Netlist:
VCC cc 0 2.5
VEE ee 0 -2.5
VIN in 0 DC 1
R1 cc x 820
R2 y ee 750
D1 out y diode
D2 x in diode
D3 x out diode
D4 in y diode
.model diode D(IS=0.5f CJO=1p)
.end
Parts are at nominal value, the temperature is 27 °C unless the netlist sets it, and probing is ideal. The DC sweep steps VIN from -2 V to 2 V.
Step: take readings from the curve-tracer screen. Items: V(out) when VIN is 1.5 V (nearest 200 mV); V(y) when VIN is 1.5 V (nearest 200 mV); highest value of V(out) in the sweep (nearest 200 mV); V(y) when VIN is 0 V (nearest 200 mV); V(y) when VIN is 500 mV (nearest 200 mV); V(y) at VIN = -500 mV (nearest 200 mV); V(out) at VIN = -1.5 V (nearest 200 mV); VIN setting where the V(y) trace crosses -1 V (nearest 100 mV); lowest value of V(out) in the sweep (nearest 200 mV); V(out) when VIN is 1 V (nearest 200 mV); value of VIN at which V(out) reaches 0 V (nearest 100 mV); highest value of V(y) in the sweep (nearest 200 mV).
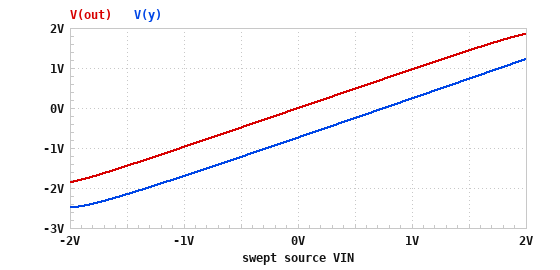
1.4 V
800 mV
1.8 V
-800 mV
-200 mV
-1.2 V
-1.4 V
-300 mV
-1.8 V
1.0 V
0 V
1.2 V
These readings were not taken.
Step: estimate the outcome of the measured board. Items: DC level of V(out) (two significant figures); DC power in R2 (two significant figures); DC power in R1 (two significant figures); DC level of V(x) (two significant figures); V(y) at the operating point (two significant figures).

970 mV
10 mW
800 µW
1.7 V
240 mV
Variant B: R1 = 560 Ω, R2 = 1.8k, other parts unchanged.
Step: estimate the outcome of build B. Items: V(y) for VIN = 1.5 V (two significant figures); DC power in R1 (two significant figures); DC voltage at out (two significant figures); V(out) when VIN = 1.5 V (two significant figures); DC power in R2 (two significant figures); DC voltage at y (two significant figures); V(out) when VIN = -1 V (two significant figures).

760 mV
1.1 mW
1.0 V
1.5 V
4.3 mW
270 mV
-940 mV
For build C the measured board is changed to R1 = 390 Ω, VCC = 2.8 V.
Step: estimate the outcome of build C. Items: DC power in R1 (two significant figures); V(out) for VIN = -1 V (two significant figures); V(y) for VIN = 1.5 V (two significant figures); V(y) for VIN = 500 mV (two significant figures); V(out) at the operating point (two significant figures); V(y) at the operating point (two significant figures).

2.9 mW
-950 mV
740 mV
-240 mV
990 mV
250 mV
